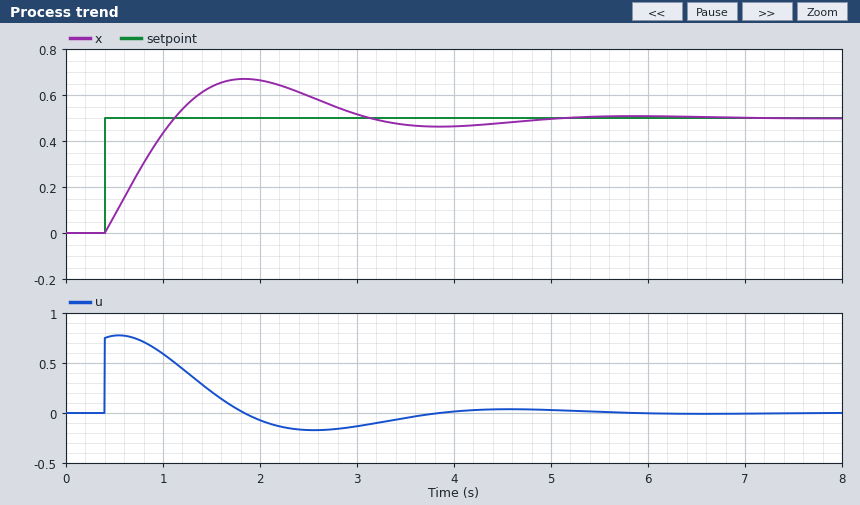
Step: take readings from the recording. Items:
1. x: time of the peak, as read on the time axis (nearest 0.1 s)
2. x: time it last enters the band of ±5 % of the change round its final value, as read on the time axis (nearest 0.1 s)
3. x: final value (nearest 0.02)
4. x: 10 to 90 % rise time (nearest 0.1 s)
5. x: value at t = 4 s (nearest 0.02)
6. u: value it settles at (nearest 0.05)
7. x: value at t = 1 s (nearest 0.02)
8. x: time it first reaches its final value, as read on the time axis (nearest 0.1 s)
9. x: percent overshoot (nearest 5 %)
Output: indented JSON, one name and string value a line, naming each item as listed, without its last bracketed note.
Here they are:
{
  "x: time of the peak, as read on the time axis": "1.8 s",
  "x: time it last enters the band of ±5 % of the change round its final value, as read on the time axis": "4.4 s",
  "x: final value": "0.50",
  "x: 10 to 90 % rise time": "0.6 s",
  "x: value at t = 4 s": "0.46",
  "u: value it settles at": "0.00",
  "x: value at t = 1 s": "0.44",
  "x: time it first reaches its final value, as read on the time axis": "1.1 s",
  "x: percent overshoot": "35 %"
}
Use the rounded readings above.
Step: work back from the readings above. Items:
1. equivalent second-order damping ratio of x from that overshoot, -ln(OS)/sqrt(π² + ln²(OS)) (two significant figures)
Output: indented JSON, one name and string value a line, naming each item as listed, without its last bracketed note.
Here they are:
{
  "equivalent second-order damping ratio of x from that overshoot, -ln(OS)/sqrt(π² + ln²(OS))": "0.32"
}
